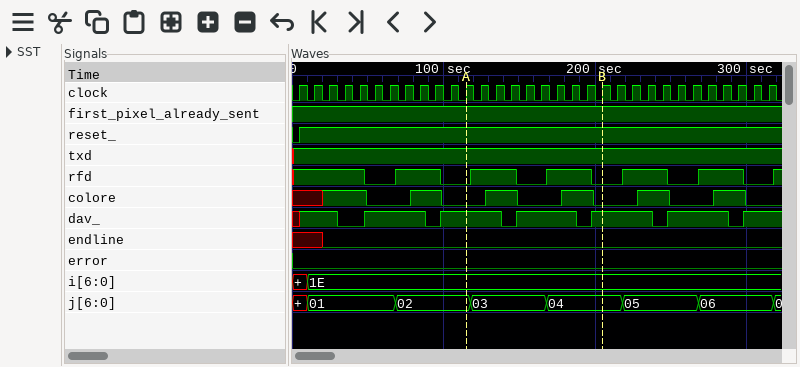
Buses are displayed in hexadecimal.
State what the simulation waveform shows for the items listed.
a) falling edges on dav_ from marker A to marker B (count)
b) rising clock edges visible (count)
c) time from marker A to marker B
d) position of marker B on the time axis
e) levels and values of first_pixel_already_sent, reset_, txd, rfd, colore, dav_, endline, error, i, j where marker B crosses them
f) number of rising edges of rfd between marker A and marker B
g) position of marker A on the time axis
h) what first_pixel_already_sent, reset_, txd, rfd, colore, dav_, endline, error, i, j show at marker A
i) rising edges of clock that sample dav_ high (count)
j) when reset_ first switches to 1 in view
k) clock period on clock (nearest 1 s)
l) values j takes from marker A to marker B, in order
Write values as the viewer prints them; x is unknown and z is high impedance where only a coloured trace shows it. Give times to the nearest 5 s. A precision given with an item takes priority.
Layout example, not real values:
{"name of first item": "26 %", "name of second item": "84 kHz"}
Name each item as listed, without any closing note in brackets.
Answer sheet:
{"falling edges on dav_ from marker A to marker B": "2", "rising clock edges visible": "32", "time from marker A to marker B": "90 s", "position of marker B on the time axis": "205 s", "levels and values of first_pixel_already_sent, reset_, txd, rfd, colore, dav_, endline, error, i, j where marker B crosses them": "first_pixel_already_sent=1, reset_=1, txd=1, rfd=0, colore=0, dav_=1, endline=0, error=0, i=1E, j=04", "number of rising edges of rfd between marker A and marker B": "2", "position of marker A on the time axis": "115 s", "what first_pixel_already_sent, reset_, txd, rfd, colore, dav_, endline, error, i, j show at marker A": "first_pixel_already_sent=1, reset_=1, txd=1, rfd=0, colore=0, dav_=1, endline=0, error=0, i=1E, j=02", "rising edges of clock that sample dav_ high": "24", "when reset_ first switches to 1 in view": "5 s", "clock period on clock": "10 s", "values j takes from marker A to marker B, in order": "02, 03, 04"}
